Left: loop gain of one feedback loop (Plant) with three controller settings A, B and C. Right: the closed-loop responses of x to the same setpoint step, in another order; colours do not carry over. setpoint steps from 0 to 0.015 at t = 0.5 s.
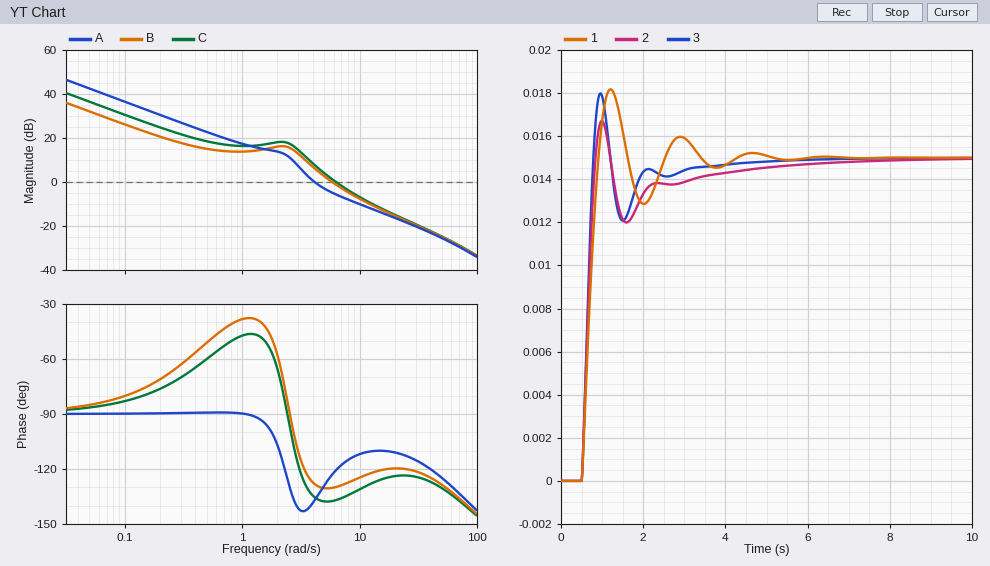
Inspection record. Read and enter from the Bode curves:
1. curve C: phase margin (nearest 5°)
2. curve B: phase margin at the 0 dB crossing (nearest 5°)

45°
50°
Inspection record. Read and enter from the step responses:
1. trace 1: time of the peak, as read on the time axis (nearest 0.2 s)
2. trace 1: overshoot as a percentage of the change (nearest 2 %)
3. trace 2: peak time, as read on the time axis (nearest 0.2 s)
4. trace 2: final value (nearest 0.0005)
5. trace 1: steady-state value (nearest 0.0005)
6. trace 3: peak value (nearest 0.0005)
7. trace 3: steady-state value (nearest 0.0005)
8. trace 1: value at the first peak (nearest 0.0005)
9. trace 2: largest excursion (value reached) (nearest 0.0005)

1.2 s
22 %
1.0 s
0.0150
0.0150
0.0180
0.0150
0.0180
0.0165
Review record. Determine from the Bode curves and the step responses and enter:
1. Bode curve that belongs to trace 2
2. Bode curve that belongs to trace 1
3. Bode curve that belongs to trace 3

B
A
C
